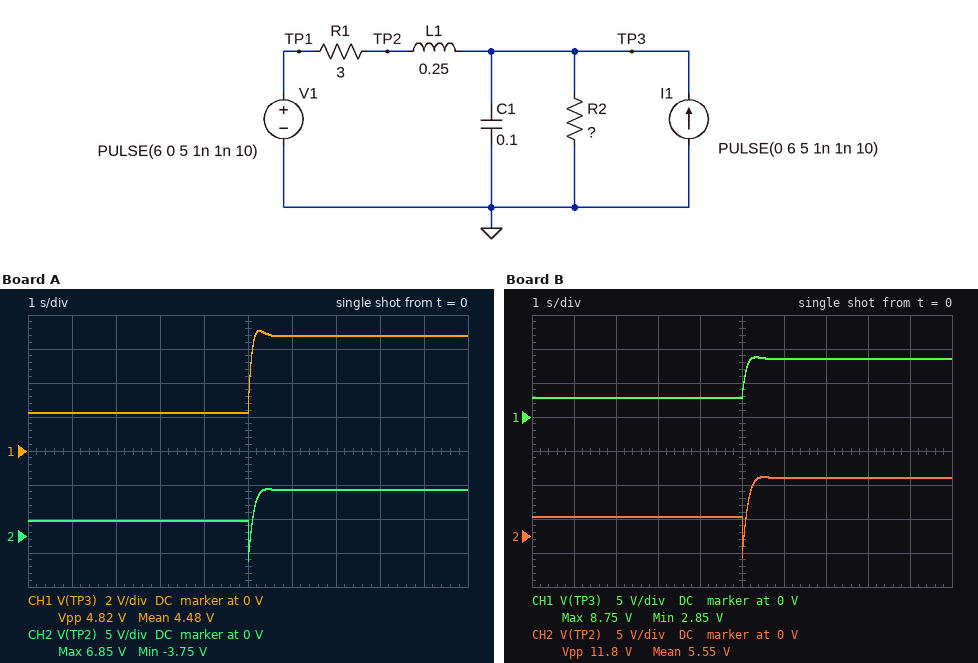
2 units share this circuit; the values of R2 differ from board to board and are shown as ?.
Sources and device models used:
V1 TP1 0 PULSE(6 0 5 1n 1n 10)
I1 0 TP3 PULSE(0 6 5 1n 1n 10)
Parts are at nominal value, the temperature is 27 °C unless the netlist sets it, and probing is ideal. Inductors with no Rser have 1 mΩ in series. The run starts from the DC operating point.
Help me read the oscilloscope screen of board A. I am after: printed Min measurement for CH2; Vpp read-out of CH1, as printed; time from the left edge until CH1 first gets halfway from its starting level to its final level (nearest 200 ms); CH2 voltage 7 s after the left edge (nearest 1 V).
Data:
-3.75 V
4.82 V
5.0 s
7 V
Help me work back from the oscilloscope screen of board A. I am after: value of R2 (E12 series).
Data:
1.8 Ω
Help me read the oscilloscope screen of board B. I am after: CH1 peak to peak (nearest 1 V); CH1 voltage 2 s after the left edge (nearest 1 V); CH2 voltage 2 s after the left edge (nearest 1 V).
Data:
6 V
3 V
3 V
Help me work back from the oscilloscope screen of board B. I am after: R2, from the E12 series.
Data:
2.7 Ω
